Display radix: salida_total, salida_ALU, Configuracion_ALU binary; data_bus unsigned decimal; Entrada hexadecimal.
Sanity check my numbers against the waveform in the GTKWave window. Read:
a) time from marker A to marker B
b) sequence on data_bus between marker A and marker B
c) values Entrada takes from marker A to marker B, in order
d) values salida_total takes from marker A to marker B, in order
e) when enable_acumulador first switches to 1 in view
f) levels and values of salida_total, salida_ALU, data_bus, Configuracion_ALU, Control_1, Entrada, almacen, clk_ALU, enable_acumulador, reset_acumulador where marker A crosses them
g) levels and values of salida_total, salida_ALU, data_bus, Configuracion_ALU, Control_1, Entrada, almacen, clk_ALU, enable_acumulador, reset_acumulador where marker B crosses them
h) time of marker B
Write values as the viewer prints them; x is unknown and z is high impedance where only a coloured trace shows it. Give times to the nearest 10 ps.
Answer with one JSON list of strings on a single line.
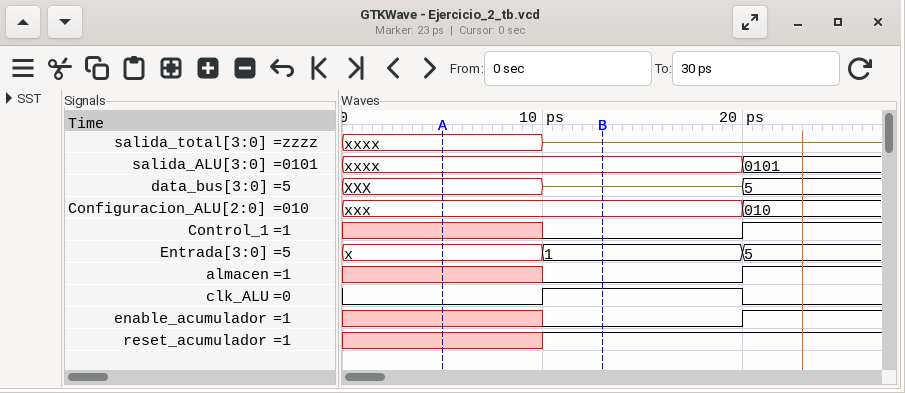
["10 ps", "XXX, z", "x, 1", "xxxx, z", "20 ps", "salida_total=xxxx, salida_ALU=xxxx, data_bus=XXX, Configuracion_ALU=xxx, Control_1=x, Entrada=x, almacen=x, clk_ALU=0, enable_acumulador=x, reset_acumulador=x", "salida_total=z, salida_ALU=xxxx, data_bus=z, Configuracion_ALU=xxx, Control_1=0, Entrada=1, almacen=0, clk_ALU=1, enable_acumulador=0, reset_acumulador=1", "10 ps"]
